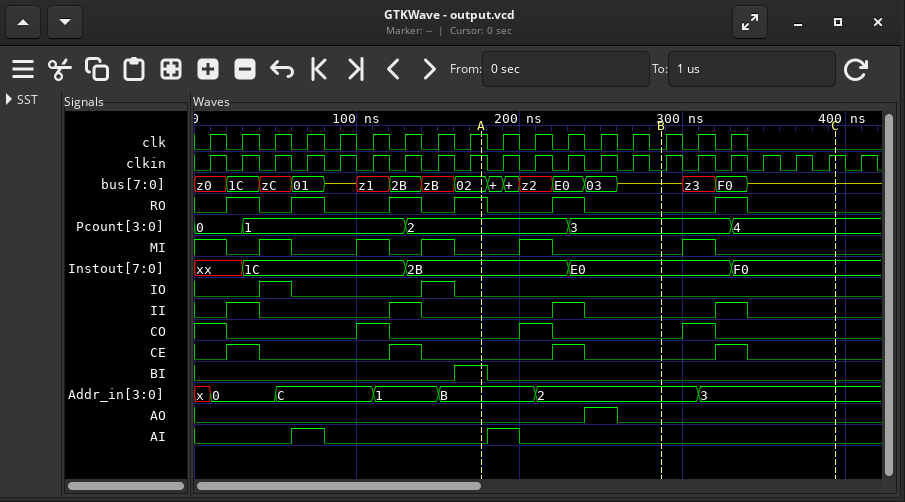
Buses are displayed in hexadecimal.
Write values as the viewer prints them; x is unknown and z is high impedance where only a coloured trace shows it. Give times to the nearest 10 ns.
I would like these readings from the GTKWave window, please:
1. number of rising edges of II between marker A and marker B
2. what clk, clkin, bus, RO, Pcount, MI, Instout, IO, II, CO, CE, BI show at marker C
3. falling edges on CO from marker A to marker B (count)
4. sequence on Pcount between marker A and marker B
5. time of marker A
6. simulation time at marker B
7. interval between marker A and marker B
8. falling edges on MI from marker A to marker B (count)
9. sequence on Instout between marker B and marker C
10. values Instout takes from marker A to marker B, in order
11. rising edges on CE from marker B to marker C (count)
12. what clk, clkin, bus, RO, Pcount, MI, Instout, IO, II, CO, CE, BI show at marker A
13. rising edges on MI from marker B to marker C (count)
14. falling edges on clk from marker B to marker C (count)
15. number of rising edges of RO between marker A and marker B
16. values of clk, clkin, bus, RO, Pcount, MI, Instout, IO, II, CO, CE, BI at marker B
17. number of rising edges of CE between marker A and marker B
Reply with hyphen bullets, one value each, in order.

- 1
- clk=0, clkin=1, bus=z, RO=0, Pcount=4, MI=0, Instout=F0, IO=0, II=0, CO=0, CE=0, BI=0
- 1
- 2, 3
- 180 ns
- 290 ns
- 110 ns
- 1
- E0, F0
- 2B, E0
- 1
- clk=1, clkin=1, bus=02, RO=1, Pcount=2, MI=0, Instout=2B, IO=0, II=0, CO=0, CE=0, BI=1
- 1
- 3
- 1
- clk=0, clkin=0, bus=z, RO=0, Pcount=3, MI=0, Instout=E0, IO=0, II=0, CO=0, CE=0, BI=0
- 1
